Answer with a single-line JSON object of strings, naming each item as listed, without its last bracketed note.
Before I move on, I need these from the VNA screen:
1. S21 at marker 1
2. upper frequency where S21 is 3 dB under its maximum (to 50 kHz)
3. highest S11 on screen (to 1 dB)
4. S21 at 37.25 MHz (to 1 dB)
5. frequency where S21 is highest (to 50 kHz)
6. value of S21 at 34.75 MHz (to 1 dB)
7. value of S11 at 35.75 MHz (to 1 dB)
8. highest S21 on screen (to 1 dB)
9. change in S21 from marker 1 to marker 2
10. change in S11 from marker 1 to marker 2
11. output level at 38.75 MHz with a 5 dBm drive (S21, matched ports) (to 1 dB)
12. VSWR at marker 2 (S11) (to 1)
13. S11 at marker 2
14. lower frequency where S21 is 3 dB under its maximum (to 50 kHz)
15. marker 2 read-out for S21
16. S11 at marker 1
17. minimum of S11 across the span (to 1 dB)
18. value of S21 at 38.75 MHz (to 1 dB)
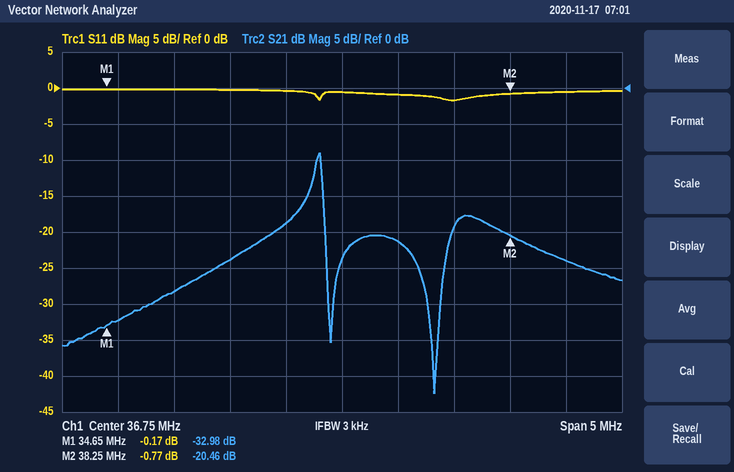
{"S21 at marker 1": "-32.98 dB", "upper frequency where S21 is 3 dB under its maximum": "36.55 MHz", "highest S11 on screen": "0 dB", "S21 at 37.25 MHz": "-21 dB", "frequency where S21 is highest": "36.55 MHz", "value of S21 at 34.75 MHz": "-32 dB", "value of S11 at 35.75 MHz": "0 dB", "highest S21 on screen": "-9 dB", "change in S21 from marker 1 to marker 2": "12.52 dB", "change in S11 from marker 1 to marker 2": "-0.60 dB", "output level at 38.75 MHz with a 5 dBm drive (S21, matched ports)": "-19 dBm", "VSWR at marker 2 (S11)": "23", "S11 at marker 2": "-0.77 dB", "lower frequency where S21 is 3 dB under its maximum": "36.50 MHz", "marker 2 read-out for S21": "-20.46 dB", "S11 at marker 1": "-0.17 dB", "minimum of S11 across the span": "-2 dB", "value of S21 at 38.75 MHz": "-24 dB"}
